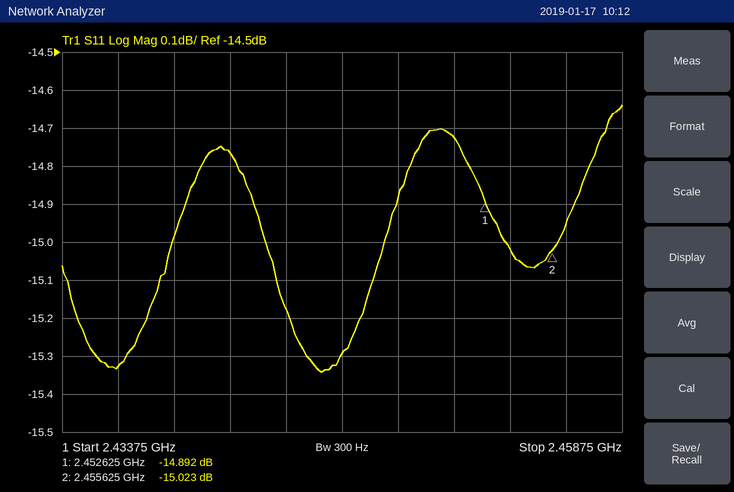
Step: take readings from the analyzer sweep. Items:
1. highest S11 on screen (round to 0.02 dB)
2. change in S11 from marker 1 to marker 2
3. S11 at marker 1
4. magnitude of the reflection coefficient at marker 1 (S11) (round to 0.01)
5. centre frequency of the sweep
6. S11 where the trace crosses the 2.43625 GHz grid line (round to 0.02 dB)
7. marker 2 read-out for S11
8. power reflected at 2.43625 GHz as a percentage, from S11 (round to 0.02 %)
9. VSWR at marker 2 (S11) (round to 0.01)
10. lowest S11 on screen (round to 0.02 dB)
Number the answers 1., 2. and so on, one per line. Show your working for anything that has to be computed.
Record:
1. -14.64 dB
2. -15.023 − (-14.892) = -0.131 dB
3. -14.892 dB
4. 10^(-14.892/20) ≈ 0.18
5. 2.44625 GHz
6. -15.32 dB
7. -15.023 dB
8. 10^(-15.32/10) ≈ 2.94 %
9. (1 + 0.1774)/(1 − 0.1774) ≈ 1.43
10. -15.34 dB
